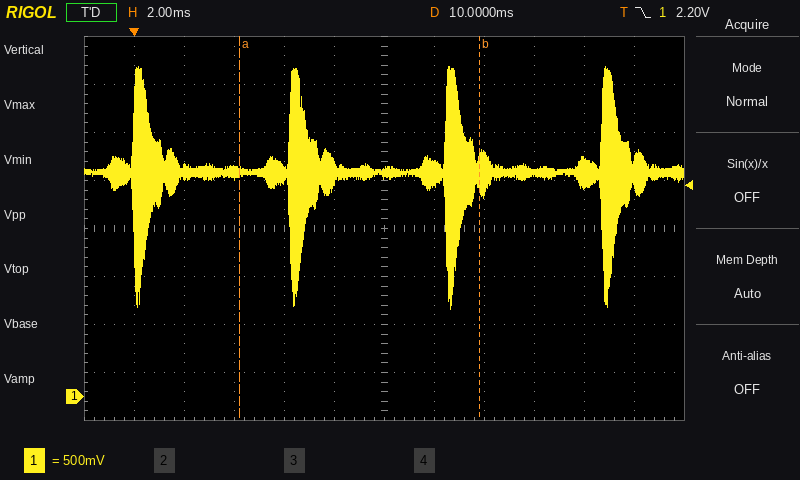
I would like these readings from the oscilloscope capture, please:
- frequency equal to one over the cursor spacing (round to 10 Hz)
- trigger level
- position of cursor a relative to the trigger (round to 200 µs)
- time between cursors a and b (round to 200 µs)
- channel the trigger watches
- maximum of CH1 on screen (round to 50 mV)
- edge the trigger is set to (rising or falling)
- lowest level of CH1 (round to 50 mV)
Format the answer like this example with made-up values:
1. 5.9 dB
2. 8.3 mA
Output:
1. 100 Hz
2. 2.20 V
3. +4.2 ms
4. 9.6 ms
5. CH1
6. 3.45 V
7. falling
8. 900 mV
